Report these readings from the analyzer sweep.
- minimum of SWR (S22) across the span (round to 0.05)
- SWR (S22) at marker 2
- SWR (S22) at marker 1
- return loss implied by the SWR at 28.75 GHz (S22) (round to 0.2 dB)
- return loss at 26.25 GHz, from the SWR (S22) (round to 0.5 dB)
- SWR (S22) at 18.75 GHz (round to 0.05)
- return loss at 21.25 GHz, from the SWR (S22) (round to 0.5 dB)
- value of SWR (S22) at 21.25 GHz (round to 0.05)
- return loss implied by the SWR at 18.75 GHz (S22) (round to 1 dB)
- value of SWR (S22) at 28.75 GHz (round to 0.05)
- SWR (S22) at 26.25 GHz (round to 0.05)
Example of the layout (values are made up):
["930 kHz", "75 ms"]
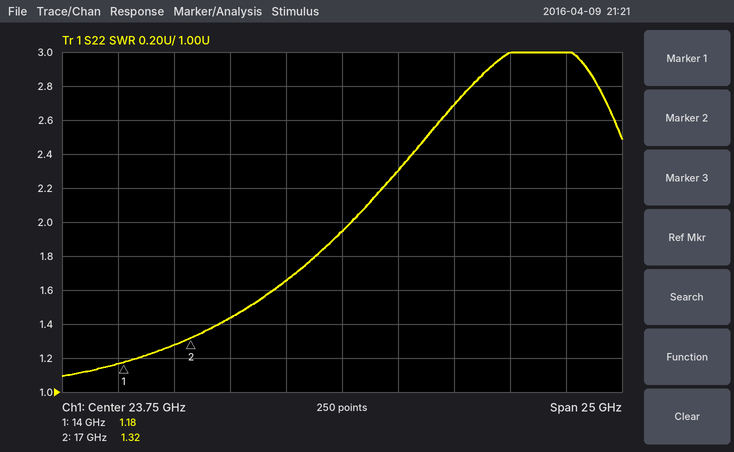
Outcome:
["1.10", "1.32", "1.18", "6.8 dB", "8.0 dB", "1.45", "12.0 dB", "1.65", "15 dB", "2.70", "2.30"]
